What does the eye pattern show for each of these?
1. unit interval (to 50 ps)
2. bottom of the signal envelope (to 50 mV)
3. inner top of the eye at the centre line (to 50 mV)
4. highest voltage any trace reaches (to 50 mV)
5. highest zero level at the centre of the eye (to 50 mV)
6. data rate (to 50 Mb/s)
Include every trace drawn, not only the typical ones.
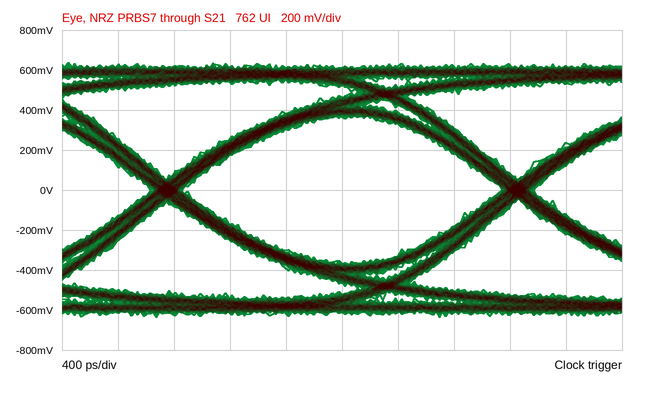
2.50 ns
-650 mV
350 mV
650 mV
-350 mV
400 Mb/s
